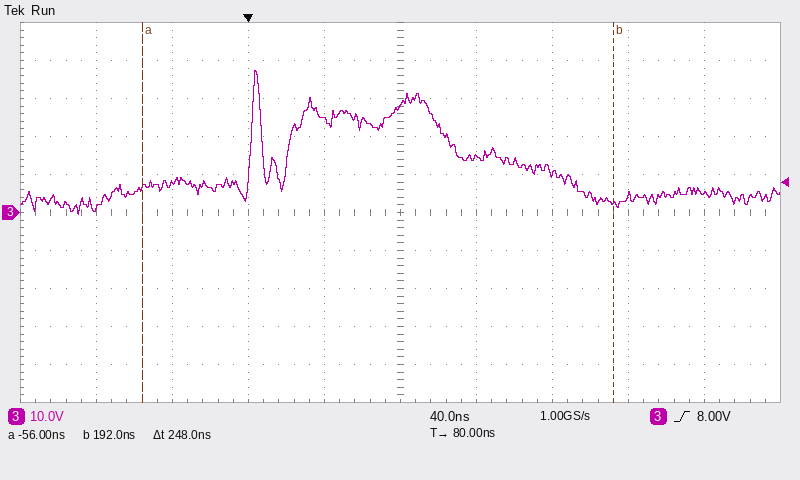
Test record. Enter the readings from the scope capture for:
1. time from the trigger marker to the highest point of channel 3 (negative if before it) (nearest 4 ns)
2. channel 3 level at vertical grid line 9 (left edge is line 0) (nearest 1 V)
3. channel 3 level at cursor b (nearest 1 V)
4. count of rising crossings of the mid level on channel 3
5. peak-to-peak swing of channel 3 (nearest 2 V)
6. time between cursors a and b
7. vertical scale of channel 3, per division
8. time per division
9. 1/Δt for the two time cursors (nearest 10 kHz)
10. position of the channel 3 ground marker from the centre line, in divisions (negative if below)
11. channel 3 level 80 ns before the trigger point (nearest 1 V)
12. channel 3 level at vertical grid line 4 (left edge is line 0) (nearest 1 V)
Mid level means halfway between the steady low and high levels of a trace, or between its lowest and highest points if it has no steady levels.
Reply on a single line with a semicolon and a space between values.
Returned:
+4 ns; 5 V; 2 V; 2; 38 V; 248 ns; 10 V; 40 ns; 4.03 MHz; 0.0 div; 1 V; 24 V
